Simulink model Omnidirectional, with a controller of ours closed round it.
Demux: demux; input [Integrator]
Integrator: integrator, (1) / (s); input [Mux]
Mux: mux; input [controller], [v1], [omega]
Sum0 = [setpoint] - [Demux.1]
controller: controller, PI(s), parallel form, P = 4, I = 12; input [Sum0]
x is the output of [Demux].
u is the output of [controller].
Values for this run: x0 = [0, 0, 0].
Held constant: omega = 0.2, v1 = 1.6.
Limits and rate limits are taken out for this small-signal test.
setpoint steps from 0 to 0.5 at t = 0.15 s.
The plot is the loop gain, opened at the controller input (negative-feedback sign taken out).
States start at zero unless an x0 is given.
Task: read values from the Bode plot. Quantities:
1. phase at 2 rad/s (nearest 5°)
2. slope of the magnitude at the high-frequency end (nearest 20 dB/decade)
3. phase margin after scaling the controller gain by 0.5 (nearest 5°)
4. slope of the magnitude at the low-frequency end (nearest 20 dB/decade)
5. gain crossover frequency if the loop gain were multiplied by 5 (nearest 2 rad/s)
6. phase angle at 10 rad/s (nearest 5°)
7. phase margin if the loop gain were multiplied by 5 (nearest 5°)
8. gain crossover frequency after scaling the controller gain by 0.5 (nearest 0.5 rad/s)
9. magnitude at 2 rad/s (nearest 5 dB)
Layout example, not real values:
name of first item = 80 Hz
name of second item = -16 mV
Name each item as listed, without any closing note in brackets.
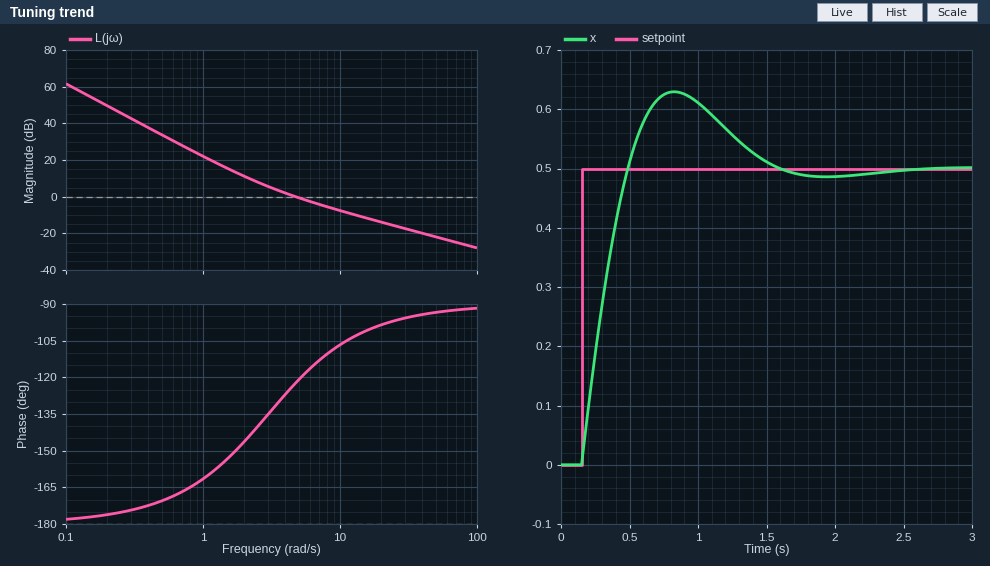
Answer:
phase at 2 rad/s = -145°
slope of the magnitude at the high-frequency end = -20 dB/decade
phase margin after scaling the controller gain by 0.5 = 45°
slope of the magnitude at the low-frequency end = -40 dB/decade
gain crossover frequency if the loop gain were multiplied by 5 = 20 rad/s
phase angle at 10 rad/s = -105°
phase margin if the loop gain were multiplied by 5 = 80°
gain crossover frequency after scaling the controller gain by 0.5 = 3.0 rad/s
magnitude at 2 rad/s = 10 dB
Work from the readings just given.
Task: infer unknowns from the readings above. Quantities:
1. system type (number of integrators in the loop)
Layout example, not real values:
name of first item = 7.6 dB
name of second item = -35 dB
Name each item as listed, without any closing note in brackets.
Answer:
system type = 2
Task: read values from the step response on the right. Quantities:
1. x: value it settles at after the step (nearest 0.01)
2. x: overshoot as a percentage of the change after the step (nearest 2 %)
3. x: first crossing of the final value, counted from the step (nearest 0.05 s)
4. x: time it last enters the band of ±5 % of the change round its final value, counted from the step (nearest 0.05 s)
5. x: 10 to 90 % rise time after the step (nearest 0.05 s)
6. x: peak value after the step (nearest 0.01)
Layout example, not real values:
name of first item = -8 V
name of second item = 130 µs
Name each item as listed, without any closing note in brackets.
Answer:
x: value it settles at after the step = 0.50
x: overshoot as a percentage of the change after the step = 26 %
x: first crossing of the final value, counted from the step = 0.35 s
x: time it last enters the band of ±5 % of the change round its final value, counted from the step = 1.25 s
x: 10 to 90 % rise time after the step = 0.25 s
x: peak value after the step = 0.63
